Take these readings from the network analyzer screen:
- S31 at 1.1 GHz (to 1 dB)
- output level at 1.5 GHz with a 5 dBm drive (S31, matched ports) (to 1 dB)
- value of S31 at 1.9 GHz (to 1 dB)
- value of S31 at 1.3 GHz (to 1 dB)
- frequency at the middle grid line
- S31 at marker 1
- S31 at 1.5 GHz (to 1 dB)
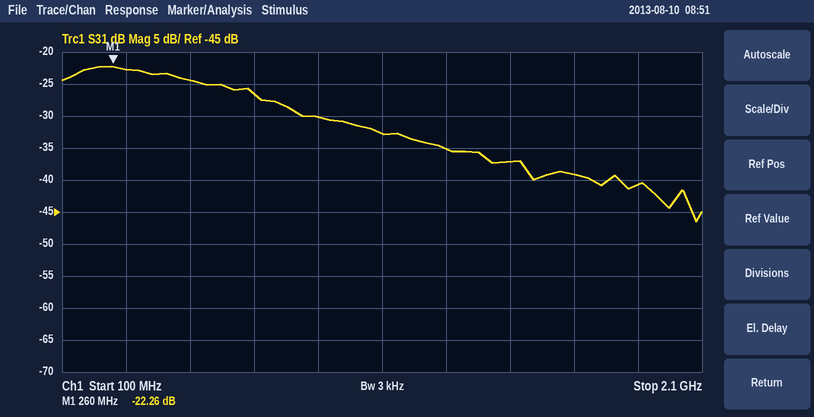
-33 dB
-32 dBm
-41 dB
-35 dB
1.1 GHz
-22.26 dB
-37 dB
